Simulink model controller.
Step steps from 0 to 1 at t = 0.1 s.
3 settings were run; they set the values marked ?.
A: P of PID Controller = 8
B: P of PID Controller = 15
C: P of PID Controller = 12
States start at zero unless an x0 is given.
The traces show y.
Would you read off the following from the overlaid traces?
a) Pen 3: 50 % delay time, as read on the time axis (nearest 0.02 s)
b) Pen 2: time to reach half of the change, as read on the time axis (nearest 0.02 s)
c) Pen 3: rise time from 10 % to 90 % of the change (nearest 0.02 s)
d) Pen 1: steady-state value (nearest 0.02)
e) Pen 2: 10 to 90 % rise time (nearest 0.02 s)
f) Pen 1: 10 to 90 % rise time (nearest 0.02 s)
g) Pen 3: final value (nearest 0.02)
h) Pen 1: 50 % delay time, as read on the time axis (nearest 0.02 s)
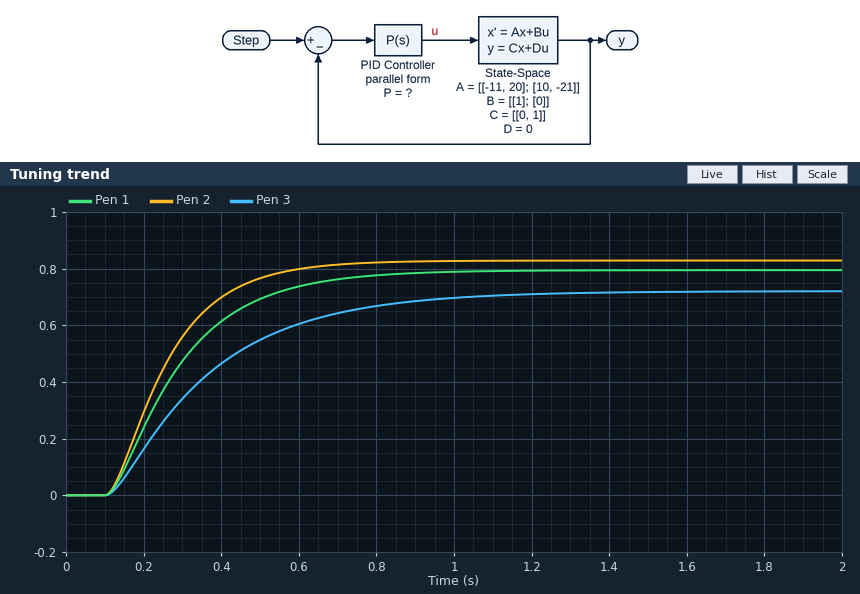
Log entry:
0.32 s
0.24 s
0.56 s
0.80
0.32 s
0.40 s
0.72
0.26 s
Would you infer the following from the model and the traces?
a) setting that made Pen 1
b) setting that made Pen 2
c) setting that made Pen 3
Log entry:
C
B
A
